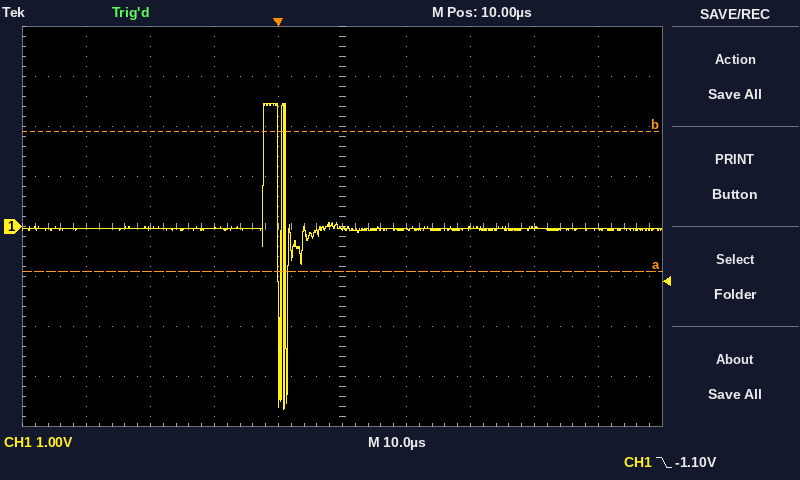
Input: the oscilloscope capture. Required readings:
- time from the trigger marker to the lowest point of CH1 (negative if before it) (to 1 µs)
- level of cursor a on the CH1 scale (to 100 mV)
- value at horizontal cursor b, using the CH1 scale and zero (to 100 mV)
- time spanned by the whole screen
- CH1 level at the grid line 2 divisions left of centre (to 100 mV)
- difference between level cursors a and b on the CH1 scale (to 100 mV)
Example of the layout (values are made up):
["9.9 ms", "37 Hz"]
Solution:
["+1 µs", "-900 mV", "1.9 V", "100 µs", "0.0 V", "2.8 V"]
